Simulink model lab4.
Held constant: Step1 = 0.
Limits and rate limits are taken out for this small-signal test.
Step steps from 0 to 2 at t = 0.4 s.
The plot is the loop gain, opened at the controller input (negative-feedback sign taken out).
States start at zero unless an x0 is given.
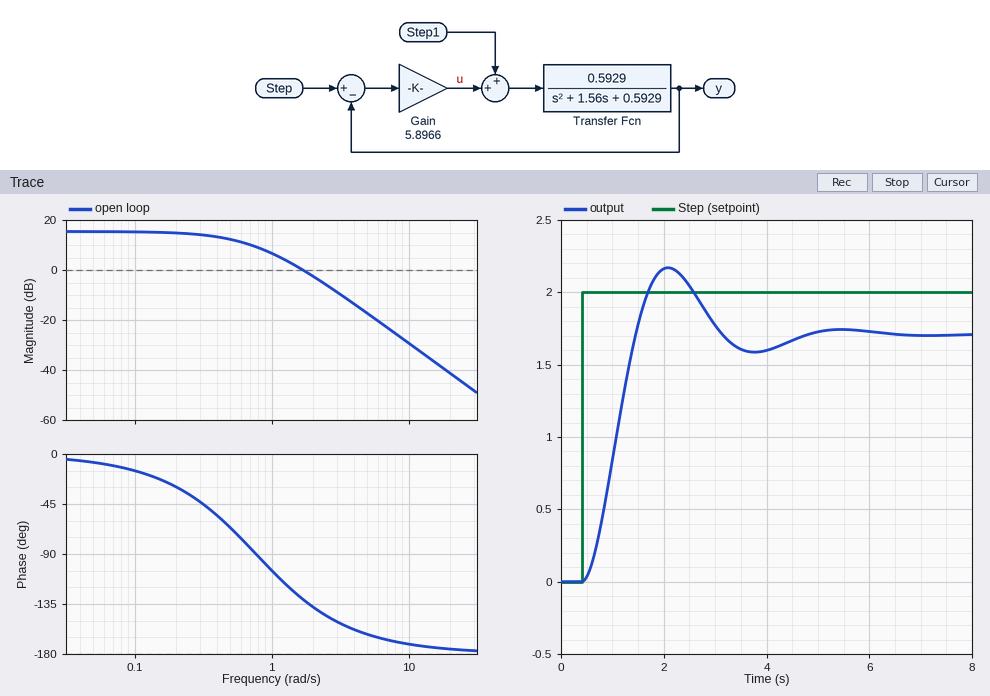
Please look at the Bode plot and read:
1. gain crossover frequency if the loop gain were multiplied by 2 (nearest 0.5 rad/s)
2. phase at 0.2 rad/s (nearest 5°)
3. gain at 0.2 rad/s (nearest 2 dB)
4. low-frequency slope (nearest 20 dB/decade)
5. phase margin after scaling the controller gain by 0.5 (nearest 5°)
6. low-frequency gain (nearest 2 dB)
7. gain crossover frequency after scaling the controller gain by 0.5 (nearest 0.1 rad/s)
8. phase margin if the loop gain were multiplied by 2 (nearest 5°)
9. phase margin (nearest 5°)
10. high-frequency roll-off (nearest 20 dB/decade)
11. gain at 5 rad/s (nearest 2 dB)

2.5 rad/s
-30°
14 dB
0 dB/decade
70°
16 dB
1.1 rad/s
35°
50°
-40 dB/decade
-18 dB
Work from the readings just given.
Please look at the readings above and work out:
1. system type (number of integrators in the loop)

0
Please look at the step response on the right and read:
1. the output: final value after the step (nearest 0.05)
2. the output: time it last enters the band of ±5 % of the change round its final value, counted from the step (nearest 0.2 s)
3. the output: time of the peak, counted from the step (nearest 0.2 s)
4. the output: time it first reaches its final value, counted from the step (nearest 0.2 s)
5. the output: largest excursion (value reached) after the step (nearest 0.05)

1.70
3.8 s
1.6 s
1.0 s
2.15
